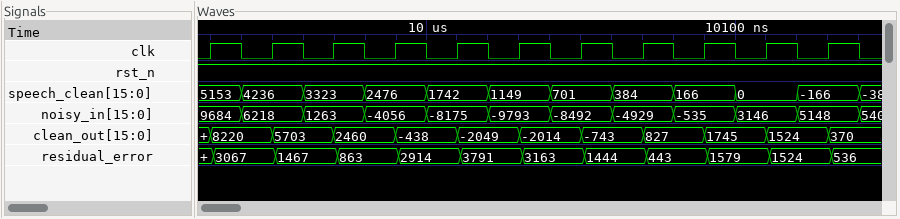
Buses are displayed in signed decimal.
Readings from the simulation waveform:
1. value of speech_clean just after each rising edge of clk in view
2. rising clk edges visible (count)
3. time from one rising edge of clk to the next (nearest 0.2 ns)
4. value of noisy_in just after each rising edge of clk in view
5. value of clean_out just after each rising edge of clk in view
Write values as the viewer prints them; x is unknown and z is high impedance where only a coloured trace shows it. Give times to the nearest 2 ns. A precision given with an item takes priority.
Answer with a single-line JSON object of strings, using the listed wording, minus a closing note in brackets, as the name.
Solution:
{"value of speech_clean just after each rising edge of clk in view": "5153, 4236, 3323, 2476, 1742, 1149, 701, 384, 166, 0, -166", "rising clk edges visible": "11", "time from one rising edge of clk to the next": "20 ns", "value of noisy_in just after each rising edge of clk in view": "9684, 6218, 1263, -4056, -8175, -9793, -8492, -4929, -535, 3146, 5148", "value of clean_out just after each rising edge of clk in view": "8220, 5703, 2460, -438, -2049, -2014, -743, 827, 1745, 1524, 370"}
